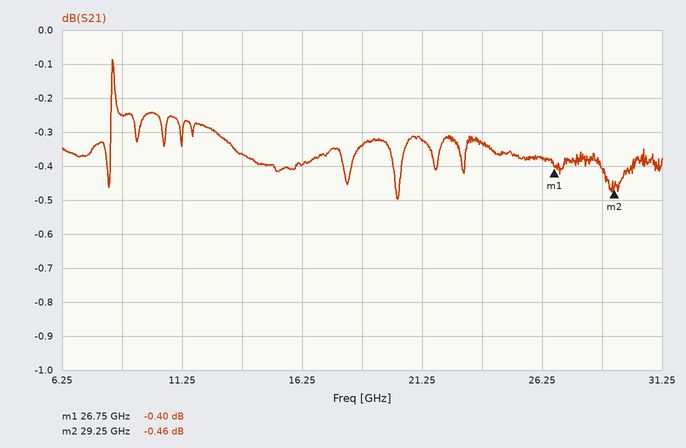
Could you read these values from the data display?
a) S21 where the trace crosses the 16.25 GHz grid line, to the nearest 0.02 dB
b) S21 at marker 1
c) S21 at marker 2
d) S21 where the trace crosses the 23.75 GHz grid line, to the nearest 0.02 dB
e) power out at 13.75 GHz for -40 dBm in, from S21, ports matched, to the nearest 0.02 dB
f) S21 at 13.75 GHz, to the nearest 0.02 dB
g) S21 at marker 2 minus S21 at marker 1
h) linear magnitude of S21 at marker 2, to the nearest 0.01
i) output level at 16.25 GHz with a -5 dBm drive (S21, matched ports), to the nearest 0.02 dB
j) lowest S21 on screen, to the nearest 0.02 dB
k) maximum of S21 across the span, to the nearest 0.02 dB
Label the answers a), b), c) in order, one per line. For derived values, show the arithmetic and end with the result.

a) -0.40 dB
b) -0.40 dB
c) -0.46 dB
d) -0.34 dB
e) -40 dBm + (-0.36 dB) = -40.36 dBm
f) -0.36 dB
g) -0.46 − (-0.4) = -0.06 dB
h) 10^(-0.46/20) ≈ 0.95
i) -5 dBm + (-0.40 dB) = -5.40 dBm
j) -0.50 dB
k) -0.08 dB
